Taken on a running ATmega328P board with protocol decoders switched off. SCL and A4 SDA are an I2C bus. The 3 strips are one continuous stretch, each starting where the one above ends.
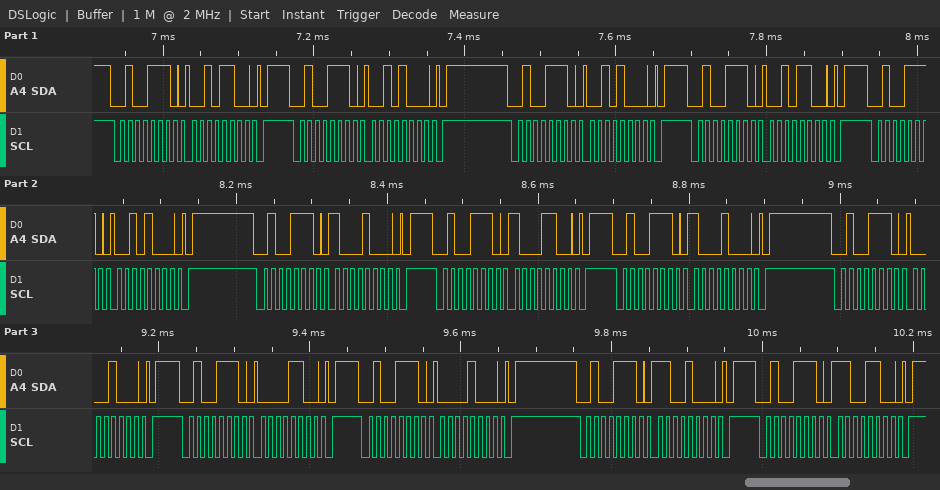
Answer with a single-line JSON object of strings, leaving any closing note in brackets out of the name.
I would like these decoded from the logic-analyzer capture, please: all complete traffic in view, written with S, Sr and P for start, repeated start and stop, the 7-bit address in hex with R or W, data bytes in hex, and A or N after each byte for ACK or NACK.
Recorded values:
{"all complete traffic in view, written with S, Sr and P for start, repeated start and stop, the 7-bit address in hex with R or W, data bytes in hex, and A or N after each byte for ACK or NACK": "S 27W A 2C A P S 27W A 28 A P S 27W A 28 A P S 27W A 2C A P S 27W A 28 A P S 27W A 88 A P S 27W A 8C A P S 27W A 88 A P S 27W A 08 A P S 27W A 0C A P S 27W A 08 A P S 27W A C8 A P S 27W A CC A P"}
